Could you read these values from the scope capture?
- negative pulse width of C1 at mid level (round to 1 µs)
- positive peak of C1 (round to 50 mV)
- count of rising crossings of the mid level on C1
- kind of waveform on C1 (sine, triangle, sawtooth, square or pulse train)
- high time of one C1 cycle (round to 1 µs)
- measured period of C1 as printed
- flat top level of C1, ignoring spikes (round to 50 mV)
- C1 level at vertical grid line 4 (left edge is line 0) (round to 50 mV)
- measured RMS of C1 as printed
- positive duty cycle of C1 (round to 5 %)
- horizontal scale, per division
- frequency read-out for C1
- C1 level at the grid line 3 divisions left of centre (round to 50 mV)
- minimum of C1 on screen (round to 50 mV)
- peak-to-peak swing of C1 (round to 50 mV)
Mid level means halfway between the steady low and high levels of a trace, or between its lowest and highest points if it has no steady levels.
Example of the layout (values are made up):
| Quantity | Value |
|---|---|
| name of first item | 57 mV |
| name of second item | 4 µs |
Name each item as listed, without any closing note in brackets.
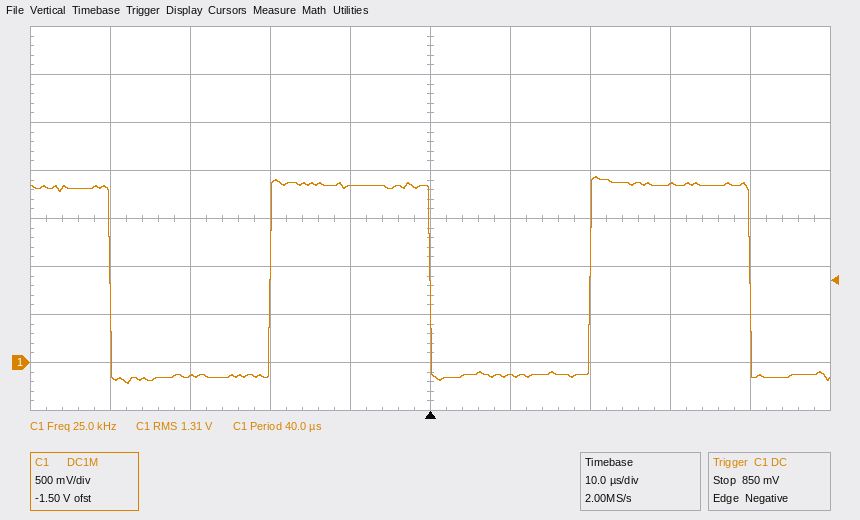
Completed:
| Quantity | Value |
|---|---|
| negative pulse width of C1 at mid level | 20 µs |
| positive peak of C1 | 1.95 V |
| count of rising crossings of the mid level on C1 | 2 |
| kind of waveform on C1 | square |
| high time of one C1 cycle | 20 µs |
| measured period of C1 as printed | 40.0 µs |
| flat top level of C1, ignoring spikes | 1.85 V |
| C1 level at vertical grid line 4 (left edge is line 0) | 1.85 V |
| measured RMS of C1 as printed | 1.31 V |
| positive duty cycle of C1 | 50 % |
| horizontal scale, per division | 10 µs |
| frequency read-out for C1 | 25.0 kHz |
| C1 level at the grid line 3 divisions left of centre | -150 mV |
| minimum of C1 on screen | -200 mV |
| peak-to-peak swing of C1 | 2.15 V |
